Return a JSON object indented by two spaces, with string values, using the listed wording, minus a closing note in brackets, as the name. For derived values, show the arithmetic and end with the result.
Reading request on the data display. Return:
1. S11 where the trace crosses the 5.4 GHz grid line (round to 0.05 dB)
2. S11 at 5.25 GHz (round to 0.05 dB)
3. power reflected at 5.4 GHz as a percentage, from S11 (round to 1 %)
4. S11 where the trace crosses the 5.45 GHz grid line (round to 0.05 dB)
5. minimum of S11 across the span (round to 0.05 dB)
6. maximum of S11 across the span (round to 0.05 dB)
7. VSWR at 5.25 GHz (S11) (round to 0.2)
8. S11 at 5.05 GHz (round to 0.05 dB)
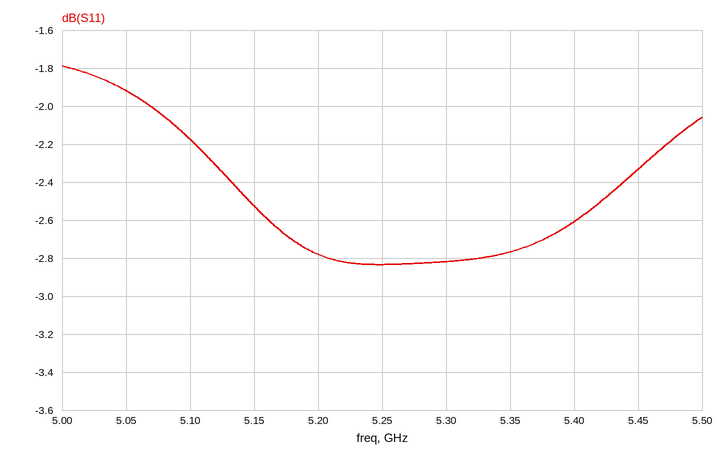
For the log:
{
  "S11 where the trace crosses the 5.4 GHz grid line": "-2.60 dB",
  "S11 at 5.25 GHz": "-2.85 dB",
  "power reflected at 5.4 GHz as a percentage, from S11": "10^(-2.6/10) ≈ 55 %",
  "S11 where the trace crosses the 5.45 GHz grid line": "-2.35 dB",
  "minimum of S11 across the span": "-2.85 dB",
  "maximum of S11 across the span": "-1.80 dB",
  "VSWR at 5.25 GHz (S11)": "|Γ| = 10^(-2.85/20) = 0.7203; VSWR = (1 + 0.7203)/(1 − 0.7203) ≈ 6.2",
  "S11 at 5.05 GHz": "-1.90 dB"
}
